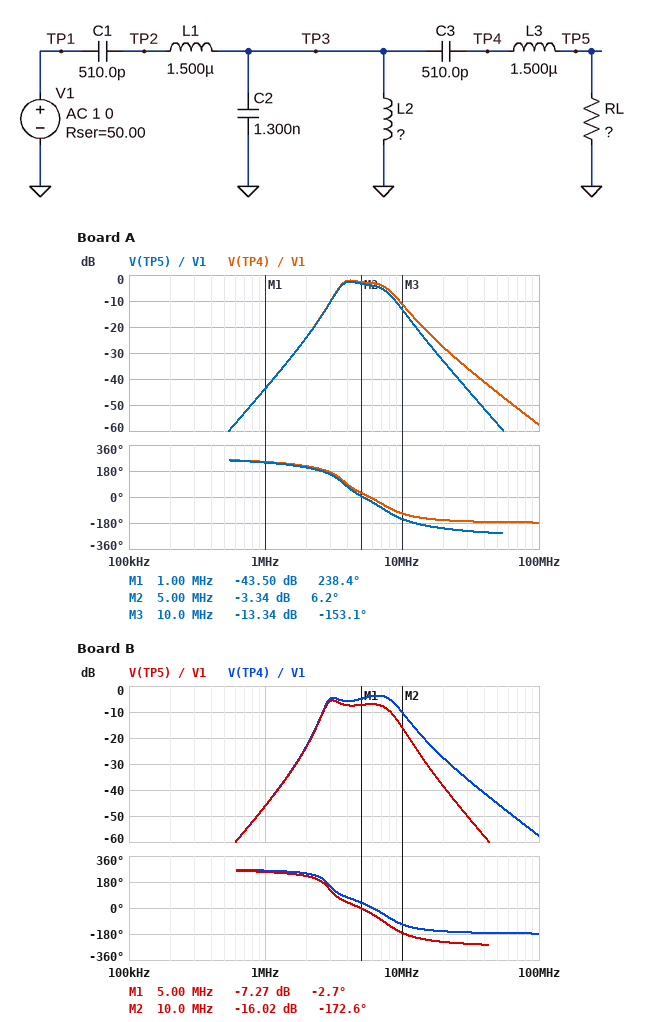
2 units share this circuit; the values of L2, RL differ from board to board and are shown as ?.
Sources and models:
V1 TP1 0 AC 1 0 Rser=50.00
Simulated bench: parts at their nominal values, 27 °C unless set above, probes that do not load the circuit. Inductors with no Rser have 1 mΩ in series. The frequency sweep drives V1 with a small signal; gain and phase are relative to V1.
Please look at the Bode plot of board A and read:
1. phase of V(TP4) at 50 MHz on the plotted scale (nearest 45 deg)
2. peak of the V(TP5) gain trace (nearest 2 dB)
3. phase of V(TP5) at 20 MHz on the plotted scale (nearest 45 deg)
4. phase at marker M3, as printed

-180 deg
-2 dB
-225 deg
-153.1 deg
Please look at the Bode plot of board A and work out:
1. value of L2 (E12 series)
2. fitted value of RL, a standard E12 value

820 nH
120 Ω
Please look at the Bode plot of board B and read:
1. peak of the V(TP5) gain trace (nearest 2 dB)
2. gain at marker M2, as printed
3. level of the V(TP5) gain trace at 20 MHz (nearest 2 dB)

-6 dB
-16.02 dB
-38 dB
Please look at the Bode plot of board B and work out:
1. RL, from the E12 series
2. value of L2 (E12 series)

56 Ω
1.2 µH
